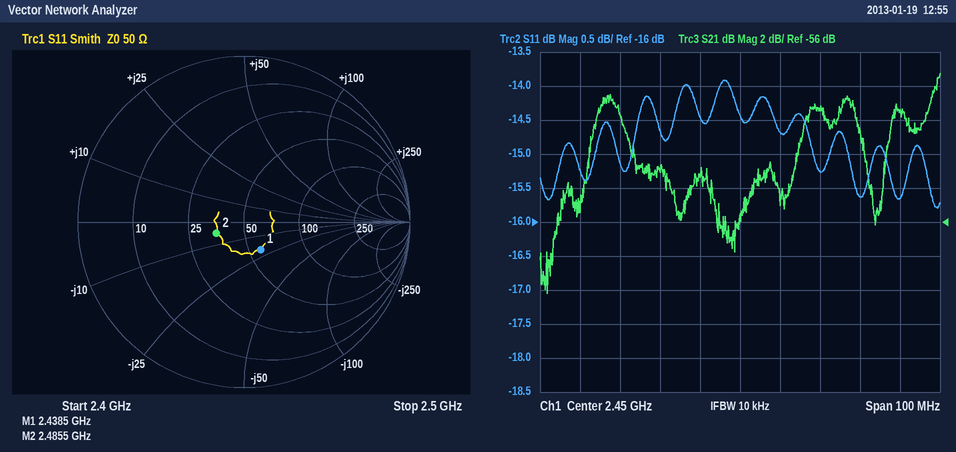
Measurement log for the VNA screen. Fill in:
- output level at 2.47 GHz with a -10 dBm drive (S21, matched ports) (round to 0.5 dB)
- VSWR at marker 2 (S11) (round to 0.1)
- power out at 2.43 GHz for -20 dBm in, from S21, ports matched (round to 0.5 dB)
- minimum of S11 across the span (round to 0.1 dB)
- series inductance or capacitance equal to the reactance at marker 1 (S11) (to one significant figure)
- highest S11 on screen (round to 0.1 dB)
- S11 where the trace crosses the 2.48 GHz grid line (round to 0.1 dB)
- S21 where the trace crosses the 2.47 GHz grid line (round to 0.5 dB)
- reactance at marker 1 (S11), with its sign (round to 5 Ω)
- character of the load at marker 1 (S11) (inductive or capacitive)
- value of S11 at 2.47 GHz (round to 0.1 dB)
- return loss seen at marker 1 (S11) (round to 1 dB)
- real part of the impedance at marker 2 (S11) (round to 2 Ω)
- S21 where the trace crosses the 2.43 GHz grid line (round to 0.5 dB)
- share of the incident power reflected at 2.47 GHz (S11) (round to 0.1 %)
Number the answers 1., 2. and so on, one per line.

1. -59.5 dBm
2. 1.4
3. -73.0 dBm
4. -15.8 dB
5. 3 pF
6. -13.9 dB
7. -15.6 dB
8. -49.5 dB
9. -20 Ω
10. capacitive
11. -15.3 dB
12. 14 dB
13. 36 Ω
14. -53.0 dB
15. 3.0 %
